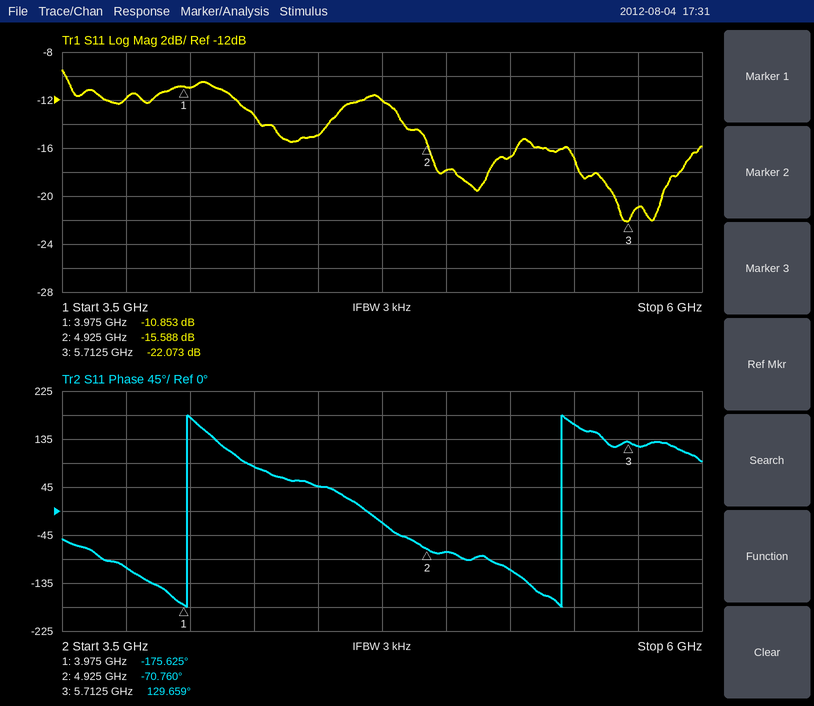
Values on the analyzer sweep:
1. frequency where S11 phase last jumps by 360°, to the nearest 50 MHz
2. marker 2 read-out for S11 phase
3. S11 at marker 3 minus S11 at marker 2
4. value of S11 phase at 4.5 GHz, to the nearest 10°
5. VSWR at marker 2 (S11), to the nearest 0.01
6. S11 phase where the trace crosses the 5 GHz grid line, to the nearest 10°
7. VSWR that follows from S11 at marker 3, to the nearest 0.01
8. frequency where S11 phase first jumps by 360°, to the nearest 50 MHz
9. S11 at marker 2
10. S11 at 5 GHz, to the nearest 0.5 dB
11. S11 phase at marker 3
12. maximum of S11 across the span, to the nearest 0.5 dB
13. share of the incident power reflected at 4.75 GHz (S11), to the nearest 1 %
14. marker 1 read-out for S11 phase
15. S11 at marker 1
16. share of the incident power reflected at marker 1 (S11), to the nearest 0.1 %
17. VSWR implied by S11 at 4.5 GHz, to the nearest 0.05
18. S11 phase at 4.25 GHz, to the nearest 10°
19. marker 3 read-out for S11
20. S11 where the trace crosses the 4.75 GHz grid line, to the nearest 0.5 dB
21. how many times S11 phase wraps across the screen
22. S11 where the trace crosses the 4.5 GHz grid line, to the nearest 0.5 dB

5.45 GHz
-70.760°
-6.485 dB
50°
1.40
-80°
1.17
4.00 GHz
-15.588 dB
-18.0 dB
129.659°
-9.5 dB
6 %
-175.625°
-10.853 dB
8.2 %
1.45
80°
-22.073 dB
-12.0 dB
2
-15.0 dB
